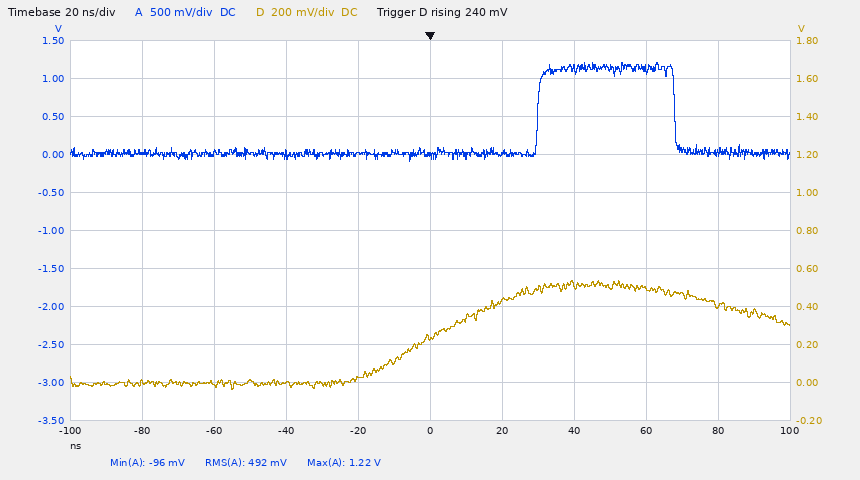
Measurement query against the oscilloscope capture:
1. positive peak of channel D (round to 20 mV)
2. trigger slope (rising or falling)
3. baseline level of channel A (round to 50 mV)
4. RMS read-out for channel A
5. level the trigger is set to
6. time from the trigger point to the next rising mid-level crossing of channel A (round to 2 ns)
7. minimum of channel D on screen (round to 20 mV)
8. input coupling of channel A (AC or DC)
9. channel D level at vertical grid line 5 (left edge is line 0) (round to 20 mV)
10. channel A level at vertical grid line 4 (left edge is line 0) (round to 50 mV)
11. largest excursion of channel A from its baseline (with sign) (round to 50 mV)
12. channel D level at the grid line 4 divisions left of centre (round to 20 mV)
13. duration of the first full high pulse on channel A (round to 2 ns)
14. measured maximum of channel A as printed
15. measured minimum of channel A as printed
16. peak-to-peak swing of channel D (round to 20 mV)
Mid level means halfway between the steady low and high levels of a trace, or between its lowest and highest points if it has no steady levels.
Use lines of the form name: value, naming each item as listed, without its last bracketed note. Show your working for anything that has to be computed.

positive peak of channel D: 540 mV
trigger slope: rising
baseline level of channel A: 0 mV
RMS read-out for channel A: 492 mV
level the trigger is set to: 240 mV
time from the trigger point to the next rising mid-level crossing of channel A: 30 ns
minimum of channel D on screen: -40 mV
input coupling of channel A: DC
channel D level at vertical grid line 5 (left edge is line 0): 240 mV
channel A level at vertical grid line 4 (left edge is line 0): 0 mV
largest excursion of channel A from its baseline (with sign): +1.20 V
channel D level at the grid line 4 divisions left of centre: 0 mV
duration of the first full high pulse on channel A: 38 ns
measured maximum of channel A as printed: 1.22 V
measured minimum of channel A as printed: -96 mV
peak-to-peak swing of channel D: 540 mV − (-40 mV) = 580 mV
